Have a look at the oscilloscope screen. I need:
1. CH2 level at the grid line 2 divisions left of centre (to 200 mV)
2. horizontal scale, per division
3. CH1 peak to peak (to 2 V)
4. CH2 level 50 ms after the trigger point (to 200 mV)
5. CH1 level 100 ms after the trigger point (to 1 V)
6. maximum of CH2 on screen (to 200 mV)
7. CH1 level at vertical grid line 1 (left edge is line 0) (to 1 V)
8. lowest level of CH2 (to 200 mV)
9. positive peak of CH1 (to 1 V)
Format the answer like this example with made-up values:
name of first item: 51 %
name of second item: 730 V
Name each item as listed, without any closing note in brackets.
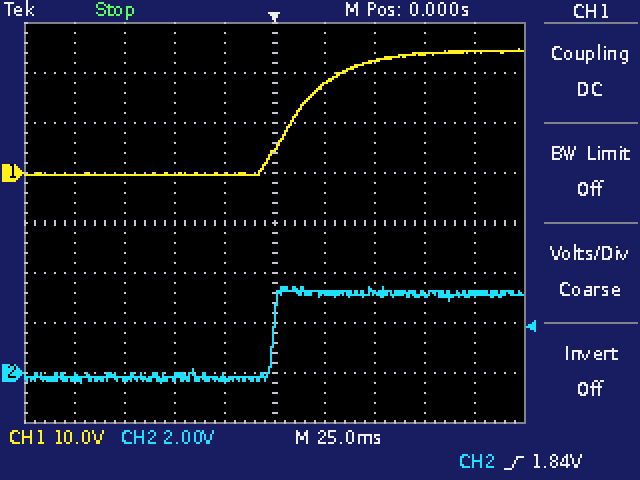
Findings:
CH2 level at the grid line 2 divisions left of centre: -200 mV
horizontal scale, per division: 25 ms
CH1 peak to peak: 26 V
CH2 level 50 ms after the trigger point: 3.2 V
CH1 level 100 ms after the trigger point: 24 V
maximum of CH2 on screen: 3.4 V
CH1 level at vertical grid line 1 (left edge is line 0): 0 V
lowest level of CH2: -400 mV
positive peak of CH1: 25 V
